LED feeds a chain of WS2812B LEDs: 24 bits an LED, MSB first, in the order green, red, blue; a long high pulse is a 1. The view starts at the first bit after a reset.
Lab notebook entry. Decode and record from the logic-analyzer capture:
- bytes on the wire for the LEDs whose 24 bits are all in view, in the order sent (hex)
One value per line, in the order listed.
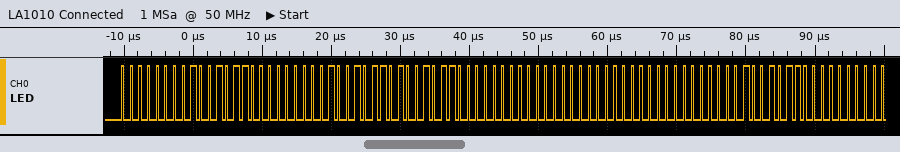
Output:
00 96 00 96 96 00 00 00 00
